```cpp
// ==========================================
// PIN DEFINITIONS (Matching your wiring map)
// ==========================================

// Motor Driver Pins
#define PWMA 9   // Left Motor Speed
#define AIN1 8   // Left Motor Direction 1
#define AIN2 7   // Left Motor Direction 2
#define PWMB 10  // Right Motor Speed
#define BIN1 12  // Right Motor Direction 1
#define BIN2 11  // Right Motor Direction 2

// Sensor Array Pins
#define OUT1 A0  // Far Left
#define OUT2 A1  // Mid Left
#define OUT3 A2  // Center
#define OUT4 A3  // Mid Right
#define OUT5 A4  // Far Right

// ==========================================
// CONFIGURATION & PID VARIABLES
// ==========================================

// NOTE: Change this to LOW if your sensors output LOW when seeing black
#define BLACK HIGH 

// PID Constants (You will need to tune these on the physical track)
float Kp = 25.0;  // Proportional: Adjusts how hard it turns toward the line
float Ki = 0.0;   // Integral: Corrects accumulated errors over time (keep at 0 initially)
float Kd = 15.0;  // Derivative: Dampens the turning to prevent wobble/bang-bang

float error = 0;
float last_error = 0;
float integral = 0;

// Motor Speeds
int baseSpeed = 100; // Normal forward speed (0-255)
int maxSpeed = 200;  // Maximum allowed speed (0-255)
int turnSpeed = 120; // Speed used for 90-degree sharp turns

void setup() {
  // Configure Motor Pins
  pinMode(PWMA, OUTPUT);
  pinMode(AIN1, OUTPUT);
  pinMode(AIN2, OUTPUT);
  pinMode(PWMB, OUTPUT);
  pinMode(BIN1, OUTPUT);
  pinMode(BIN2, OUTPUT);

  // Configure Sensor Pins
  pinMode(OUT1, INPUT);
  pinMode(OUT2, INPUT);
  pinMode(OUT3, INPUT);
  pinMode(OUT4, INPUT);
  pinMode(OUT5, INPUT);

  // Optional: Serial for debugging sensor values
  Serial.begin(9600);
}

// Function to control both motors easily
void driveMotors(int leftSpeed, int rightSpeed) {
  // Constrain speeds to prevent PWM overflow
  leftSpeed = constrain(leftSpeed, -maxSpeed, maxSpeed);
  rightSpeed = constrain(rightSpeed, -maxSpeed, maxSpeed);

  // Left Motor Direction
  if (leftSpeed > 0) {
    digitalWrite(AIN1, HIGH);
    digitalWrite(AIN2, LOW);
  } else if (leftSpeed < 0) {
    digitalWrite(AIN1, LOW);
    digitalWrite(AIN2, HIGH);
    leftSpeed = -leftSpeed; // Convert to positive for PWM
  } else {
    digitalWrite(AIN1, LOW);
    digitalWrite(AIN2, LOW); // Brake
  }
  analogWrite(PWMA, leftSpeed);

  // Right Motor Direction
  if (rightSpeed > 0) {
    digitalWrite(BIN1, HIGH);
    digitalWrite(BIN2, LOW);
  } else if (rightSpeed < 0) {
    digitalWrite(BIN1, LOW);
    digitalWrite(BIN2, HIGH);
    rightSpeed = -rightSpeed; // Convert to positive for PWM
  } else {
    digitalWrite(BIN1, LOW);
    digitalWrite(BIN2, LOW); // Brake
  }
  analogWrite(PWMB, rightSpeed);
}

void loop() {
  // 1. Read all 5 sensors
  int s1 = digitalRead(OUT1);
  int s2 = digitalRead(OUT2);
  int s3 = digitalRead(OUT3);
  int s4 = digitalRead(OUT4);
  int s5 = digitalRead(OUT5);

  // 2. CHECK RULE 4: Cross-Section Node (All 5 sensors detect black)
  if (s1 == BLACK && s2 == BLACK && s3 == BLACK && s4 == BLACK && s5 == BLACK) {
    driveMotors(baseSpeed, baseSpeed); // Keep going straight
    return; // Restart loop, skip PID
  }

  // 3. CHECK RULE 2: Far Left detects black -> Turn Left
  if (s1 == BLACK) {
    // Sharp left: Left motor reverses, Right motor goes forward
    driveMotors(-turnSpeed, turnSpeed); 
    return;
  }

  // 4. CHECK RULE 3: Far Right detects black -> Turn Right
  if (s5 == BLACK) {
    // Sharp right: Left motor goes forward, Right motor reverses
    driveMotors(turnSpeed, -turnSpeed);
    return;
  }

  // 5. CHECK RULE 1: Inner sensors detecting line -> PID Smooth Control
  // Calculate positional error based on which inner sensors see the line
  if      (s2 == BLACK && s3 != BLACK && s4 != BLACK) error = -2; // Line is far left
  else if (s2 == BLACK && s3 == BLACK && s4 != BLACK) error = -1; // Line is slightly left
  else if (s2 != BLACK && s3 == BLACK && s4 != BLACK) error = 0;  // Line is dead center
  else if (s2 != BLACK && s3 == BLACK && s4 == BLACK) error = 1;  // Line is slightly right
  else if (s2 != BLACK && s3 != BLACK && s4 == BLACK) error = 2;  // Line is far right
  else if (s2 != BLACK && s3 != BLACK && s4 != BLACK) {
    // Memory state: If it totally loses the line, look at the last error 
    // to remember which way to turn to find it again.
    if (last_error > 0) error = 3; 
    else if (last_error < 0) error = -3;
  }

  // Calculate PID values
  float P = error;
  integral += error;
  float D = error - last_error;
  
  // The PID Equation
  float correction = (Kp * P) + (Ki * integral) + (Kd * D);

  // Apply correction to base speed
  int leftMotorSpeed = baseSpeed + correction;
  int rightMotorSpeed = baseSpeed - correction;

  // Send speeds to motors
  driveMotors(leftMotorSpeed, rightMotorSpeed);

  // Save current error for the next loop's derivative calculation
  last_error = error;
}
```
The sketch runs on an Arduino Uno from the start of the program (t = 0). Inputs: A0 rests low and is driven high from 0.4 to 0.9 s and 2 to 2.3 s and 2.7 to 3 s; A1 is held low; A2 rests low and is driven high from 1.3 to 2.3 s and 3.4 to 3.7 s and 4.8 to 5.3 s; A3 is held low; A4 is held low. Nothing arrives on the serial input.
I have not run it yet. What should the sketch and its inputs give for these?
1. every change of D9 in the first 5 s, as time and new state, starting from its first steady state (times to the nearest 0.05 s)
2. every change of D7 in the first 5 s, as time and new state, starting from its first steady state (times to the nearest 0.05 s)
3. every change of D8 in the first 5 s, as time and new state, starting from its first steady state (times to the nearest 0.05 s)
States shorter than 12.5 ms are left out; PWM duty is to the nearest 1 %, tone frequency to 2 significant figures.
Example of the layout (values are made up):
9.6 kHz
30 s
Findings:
0 s PWM 39 %; 0.4 s PWM 47 %; 0.9 s PWM 39 %; 2 s PWM 47 %; 2.3 s PWM 39 %; 2.7 s PWM 47 %; 3 s PWM 39 %
0 s low; 0.4 s high; 0.9 s low; 2 s high; 2.3 s low; 2.7 s high; 3 s low
0 s high; 0.4 s low; 0.9 s high; 2 s low; 2.3 s high; 2.7 s low; 3 s high
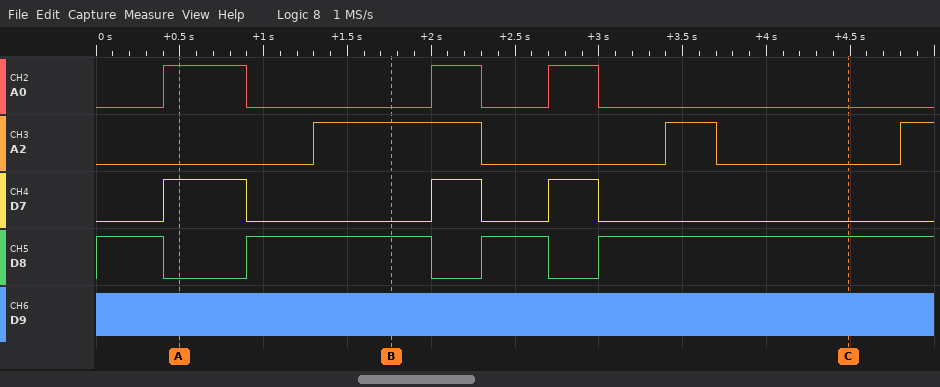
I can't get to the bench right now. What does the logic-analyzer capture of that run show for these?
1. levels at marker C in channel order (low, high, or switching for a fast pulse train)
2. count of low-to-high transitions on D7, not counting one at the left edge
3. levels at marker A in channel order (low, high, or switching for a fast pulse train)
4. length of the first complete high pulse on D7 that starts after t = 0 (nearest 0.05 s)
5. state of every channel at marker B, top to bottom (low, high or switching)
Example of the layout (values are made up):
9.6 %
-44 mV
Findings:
A0 low, A2 low, D7 low, D8 high, D9 switching
3
A0 high, A2 low, D7 high, D8 low, D9 switching
0.50 s
A0 low, A2 high, D7 low, D8 high, D9 switching
